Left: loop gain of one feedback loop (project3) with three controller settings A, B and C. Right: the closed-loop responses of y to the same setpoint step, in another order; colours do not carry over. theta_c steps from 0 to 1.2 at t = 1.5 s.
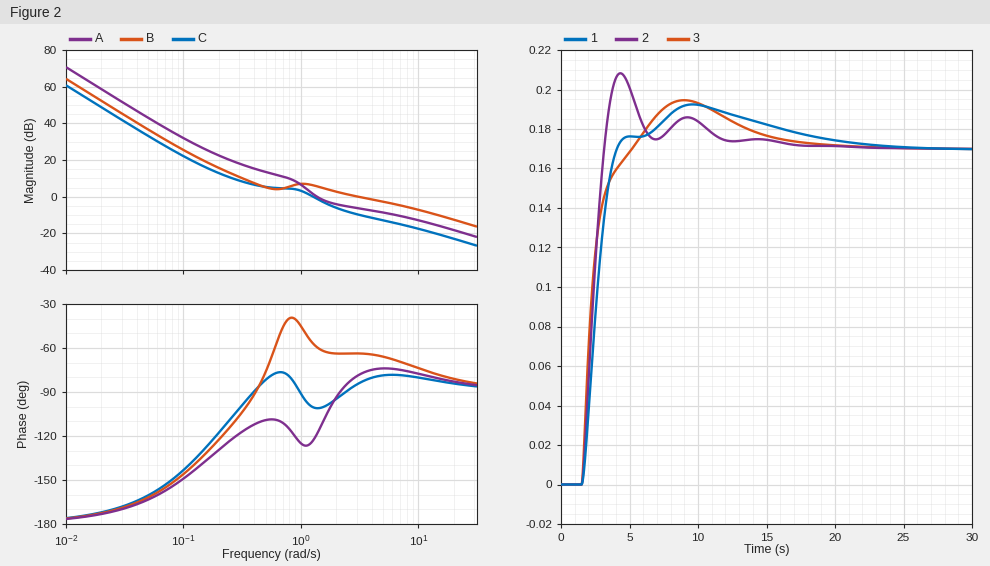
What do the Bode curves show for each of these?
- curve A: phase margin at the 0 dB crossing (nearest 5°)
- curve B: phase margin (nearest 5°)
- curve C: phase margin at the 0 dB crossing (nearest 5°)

60°
115°
80°
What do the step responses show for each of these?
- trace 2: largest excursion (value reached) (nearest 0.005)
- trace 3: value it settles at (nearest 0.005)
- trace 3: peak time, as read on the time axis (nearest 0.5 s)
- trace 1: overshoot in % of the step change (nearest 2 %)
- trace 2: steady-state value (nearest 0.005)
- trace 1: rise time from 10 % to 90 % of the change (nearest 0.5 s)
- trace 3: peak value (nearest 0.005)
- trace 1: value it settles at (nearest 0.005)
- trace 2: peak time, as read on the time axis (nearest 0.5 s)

0.210
0.170
9.0 s
14 %
0.170
1.5 s
0.195
0.170
4.5 s
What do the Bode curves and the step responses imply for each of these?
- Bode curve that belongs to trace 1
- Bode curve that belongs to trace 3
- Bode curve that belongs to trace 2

C
B
A
